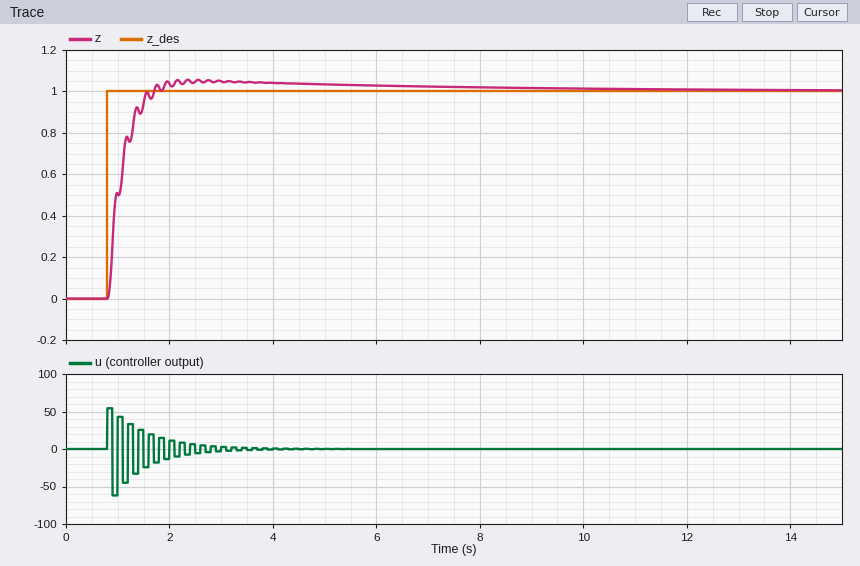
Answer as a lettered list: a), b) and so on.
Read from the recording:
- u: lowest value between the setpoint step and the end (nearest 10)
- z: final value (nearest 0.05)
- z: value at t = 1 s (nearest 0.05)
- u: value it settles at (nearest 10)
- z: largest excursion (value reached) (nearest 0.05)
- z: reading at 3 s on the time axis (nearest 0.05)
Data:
a) -60
b) 1.00
c) 0.50
d) 0
e) 1.05
f) 1.05
